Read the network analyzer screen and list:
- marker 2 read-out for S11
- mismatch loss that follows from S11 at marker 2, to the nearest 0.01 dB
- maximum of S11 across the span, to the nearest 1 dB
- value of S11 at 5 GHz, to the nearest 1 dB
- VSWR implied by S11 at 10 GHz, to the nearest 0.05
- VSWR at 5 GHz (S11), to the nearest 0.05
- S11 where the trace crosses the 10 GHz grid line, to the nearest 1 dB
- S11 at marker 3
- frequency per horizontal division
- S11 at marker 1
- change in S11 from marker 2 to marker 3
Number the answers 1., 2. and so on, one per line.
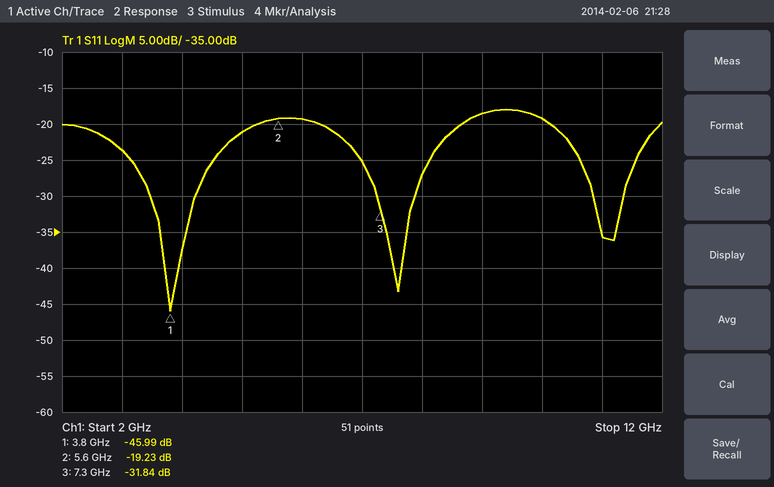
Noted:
1. -19.23 dB
2. 0.05 dB
3. -18 dB
4. -21 dB
5. 1.25
6. 1.20
7. -19 dB
8. -31.84 dB
9. 1 GHz
10. -45.99 dB
11. -12.61 dB
